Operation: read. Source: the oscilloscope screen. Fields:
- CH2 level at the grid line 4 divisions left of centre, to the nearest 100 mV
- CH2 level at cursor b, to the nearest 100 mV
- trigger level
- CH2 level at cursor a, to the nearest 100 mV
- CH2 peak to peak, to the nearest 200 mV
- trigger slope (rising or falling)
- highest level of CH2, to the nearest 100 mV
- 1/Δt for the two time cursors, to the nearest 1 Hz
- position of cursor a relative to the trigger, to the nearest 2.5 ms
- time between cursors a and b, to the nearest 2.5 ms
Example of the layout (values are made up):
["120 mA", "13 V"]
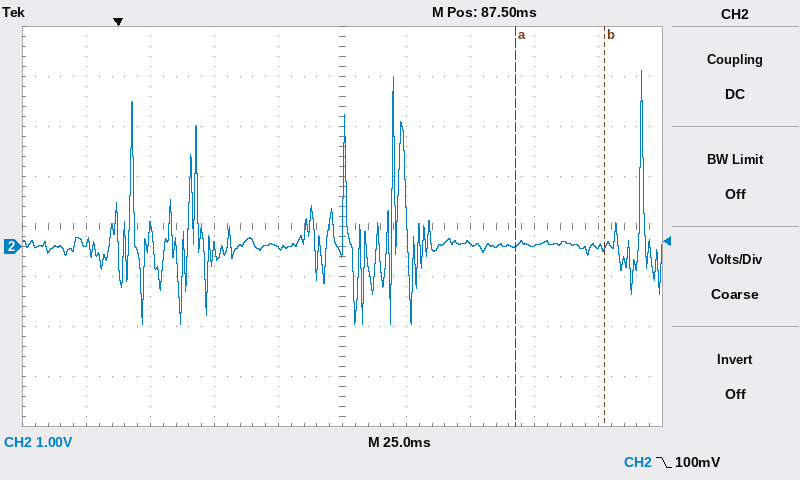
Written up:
["100 mV", "0.0 V", "100 mV", "0.0 V", "5.0 V", "falling", "3.5 V", "29 Hz", "+155.0 ms", "35.0 ms"]
